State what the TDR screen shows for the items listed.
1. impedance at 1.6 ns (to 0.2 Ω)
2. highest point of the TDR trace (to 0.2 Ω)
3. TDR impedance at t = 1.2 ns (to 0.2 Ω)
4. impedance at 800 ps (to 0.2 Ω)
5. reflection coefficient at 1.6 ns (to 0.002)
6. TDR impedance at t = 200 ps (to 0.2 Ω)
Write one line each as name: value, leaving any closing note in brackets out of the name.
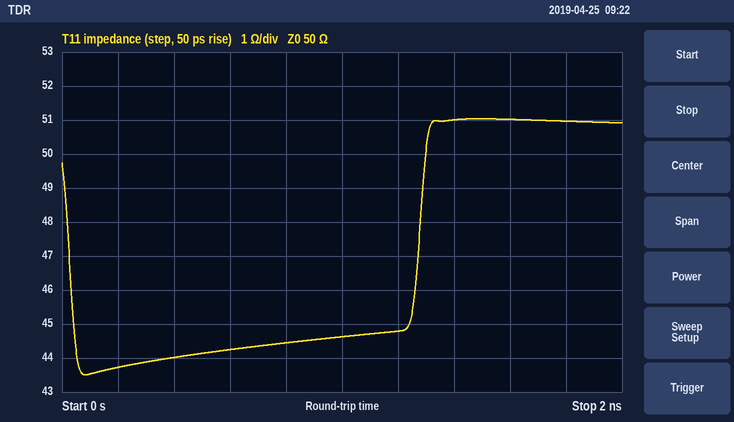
impedance at 1.6 ns: 51.0 Ω
highest point of the TDR trace: 51.0 Ω
TDR impedance at t = 1.2 ns: 44.8 Ω
impedance at 800 ps: 44.4 Ω
reflection coefficient at 1.6 ns: +0.010
TDR impedance at t = 200 ps: 43.8 Ω
